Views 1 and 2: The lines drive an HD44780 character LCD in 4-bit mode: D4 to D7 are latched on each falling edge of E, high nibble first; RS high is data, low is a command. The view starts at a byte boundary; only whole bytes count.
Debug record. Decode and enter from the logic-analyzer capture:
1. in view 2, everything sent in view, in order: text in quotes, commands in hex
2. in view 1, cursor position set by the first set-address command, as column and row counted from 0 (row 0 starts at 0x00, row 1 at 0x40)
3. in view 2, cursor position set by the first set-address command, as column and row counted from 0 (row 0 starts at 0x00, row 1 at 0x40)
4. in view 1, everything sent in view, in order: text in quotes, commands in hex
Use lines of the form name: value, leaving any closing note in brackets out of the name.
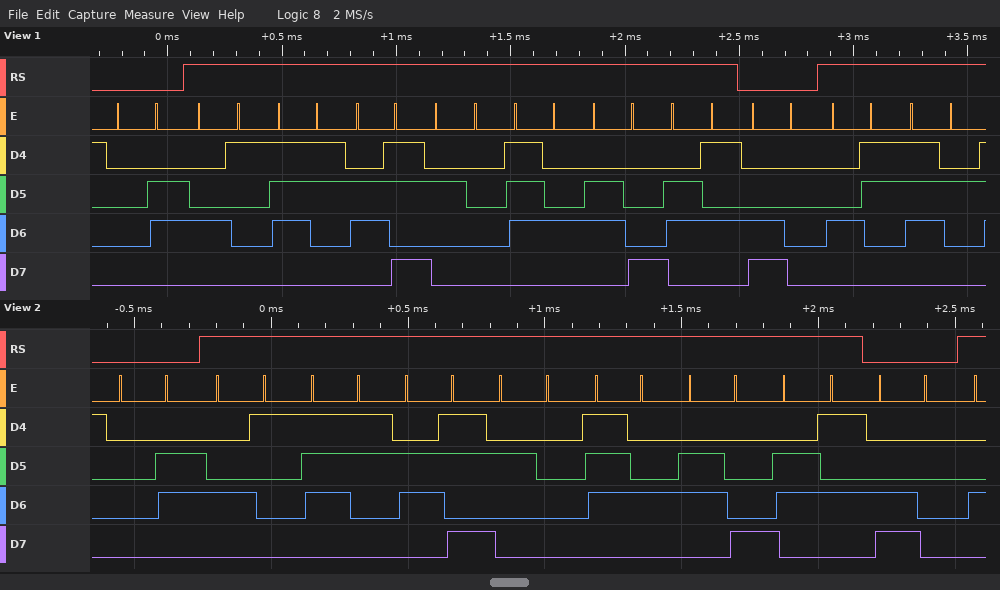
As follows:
in view 2, everything sent in view, in order: text in quotes, commands in hex: 0x06 "Ask the" 0xC0
in view 1, cursor position set by the first set-address command, as column and row counted from 0: column 0, row 1
in view 2, cursor position set by the first set-address command, as column and row counted from 0: column 0, row 1
in view 1, everything sent in view, in order: text in quotes, commands in hex: 0x06 "Ask the" 0xC0 "Cr"
